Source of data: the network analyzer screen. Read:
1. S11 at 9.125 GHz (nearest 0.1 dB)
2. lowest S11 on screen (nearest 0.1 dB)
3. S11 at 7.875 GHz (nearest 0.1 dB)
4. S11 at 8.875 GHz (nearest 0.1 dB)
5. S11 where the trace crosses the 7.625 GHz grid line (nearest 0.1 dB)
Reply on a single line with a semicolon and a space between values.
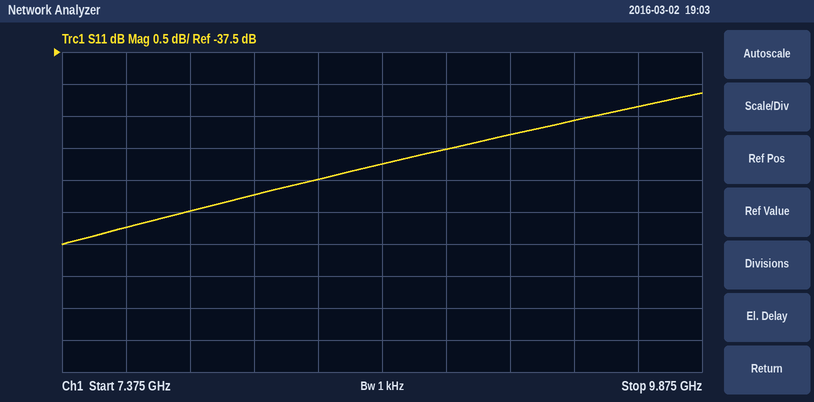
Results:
-38.8 dB; -40.5 dB; -40.0 dB; -39.0 dB; -40.2 dB
